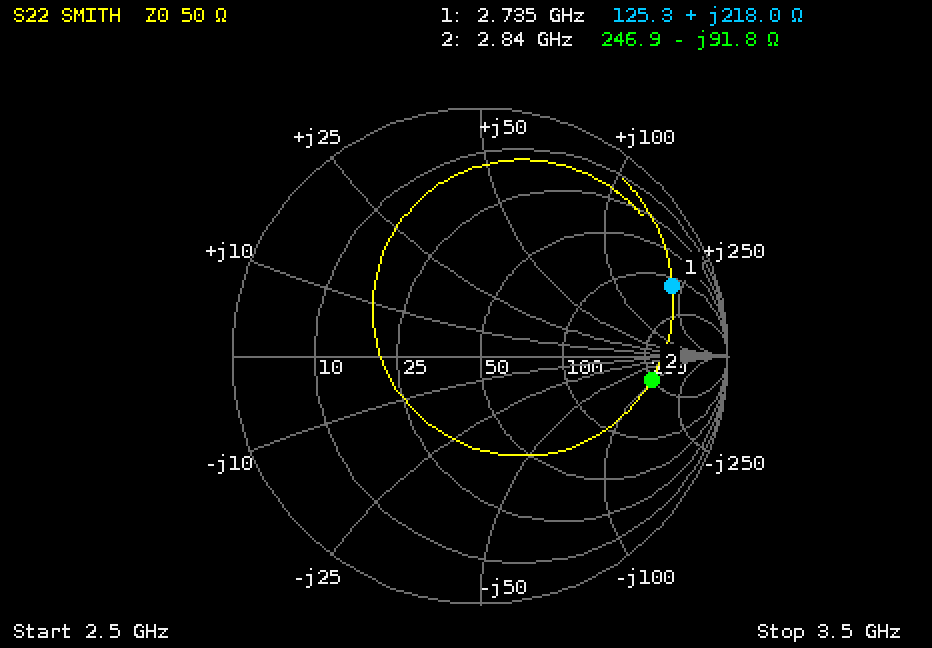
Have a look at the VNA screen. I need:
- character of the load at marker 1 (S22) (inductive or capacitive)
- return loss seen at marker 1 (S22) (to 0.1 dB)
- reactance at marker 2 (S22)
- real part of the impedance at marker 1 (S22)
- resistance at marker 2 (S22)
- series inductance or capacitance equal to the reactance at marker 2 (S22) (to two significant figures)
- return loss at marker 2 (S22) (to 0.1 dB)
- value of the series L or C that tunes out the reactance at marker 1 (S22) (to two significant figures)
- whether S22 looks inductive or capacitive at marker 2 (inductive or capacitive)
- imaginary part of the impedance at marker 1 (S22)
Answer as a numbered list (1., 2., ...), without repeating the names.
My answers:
1. inductive
2. 1.7 dB
3. -91.8 Ω
4. 125.3 Ω
5. 246.9 Ω
6. 610 fF
7. 3.1 dB
8. 270 fF
9. capacitive
10. +218.0 Ω
